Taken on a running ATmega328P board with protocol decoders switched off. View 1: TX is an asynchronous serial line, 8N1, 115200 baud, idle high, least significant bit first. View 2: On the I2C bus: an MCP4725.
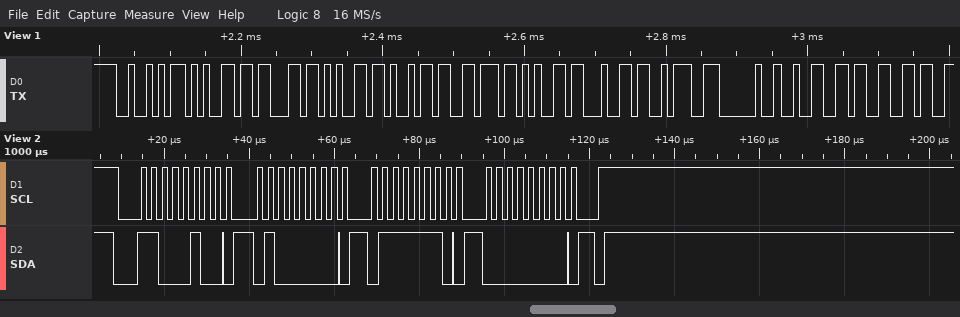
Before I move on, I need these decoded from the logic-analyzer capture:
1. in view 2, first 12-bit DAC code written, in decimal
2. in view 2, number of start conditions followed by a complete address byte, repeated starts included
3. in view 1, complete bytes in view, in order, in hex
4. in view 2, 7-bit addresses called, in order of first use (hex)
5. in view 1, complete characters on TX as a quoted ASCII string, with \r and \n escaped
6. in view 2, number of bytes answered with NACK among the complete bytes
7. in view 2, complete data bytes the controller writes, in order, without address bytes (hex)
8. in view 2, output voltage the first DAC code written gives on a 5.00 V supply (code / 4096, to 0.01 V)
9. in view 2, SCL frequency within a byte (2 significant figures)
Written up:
2016
1
0x52 0x65 0x63 0x65 0x69 0x76 0x65 0x64 0x3A 0x20 0x32 0x33
0x62
"Received: 23"
0
40 7E 00
2.46 V
400 kHz
